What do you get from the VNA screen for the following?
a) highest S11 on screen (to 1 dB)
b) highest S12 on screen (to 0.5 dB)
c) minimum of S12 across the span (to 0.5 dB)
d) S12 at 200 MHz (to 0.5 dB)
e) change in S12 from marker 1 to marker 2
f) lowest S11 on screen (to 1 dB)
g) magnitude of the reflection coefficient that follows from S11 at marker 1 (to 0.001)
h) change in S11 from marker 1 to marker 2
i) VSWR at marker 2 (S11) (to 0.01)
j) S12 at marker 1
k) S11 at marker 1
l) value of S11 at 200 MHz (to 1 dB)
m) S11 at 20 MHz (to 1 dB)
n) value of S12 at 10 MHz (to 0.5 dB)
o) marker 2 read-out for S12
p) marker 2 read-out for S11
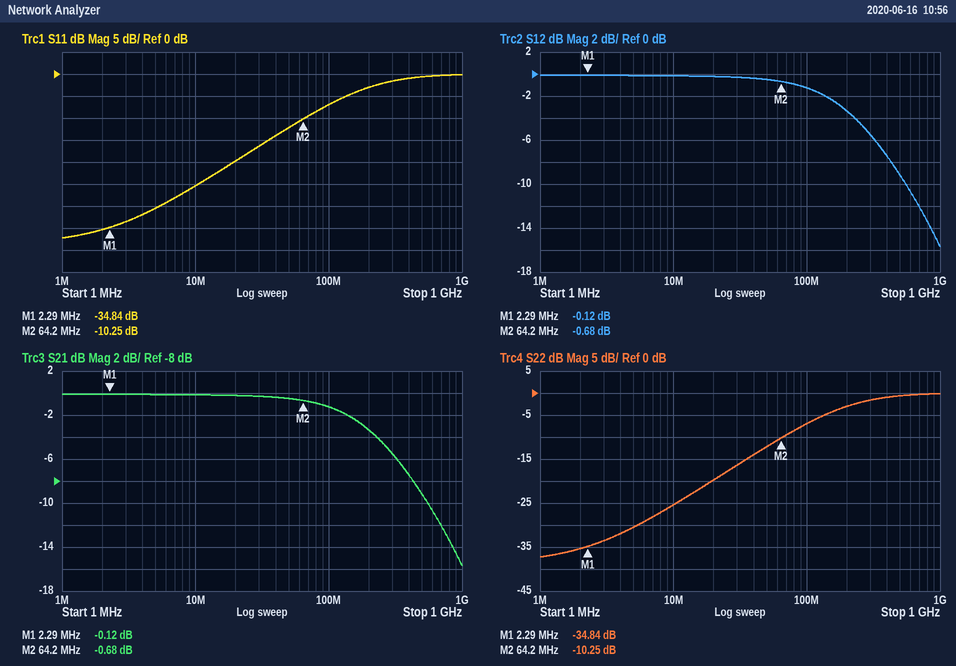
0 dB
0.0 dB
-15.5 dB
-3.5 dB
-0.56 dB
-37 dB
0.018
24.59 dB
1.89
-0.12 dB
-34.84 dB
-3 dB
-20 dB
0.0 dB
-0.68 dB
-10.25 dB
